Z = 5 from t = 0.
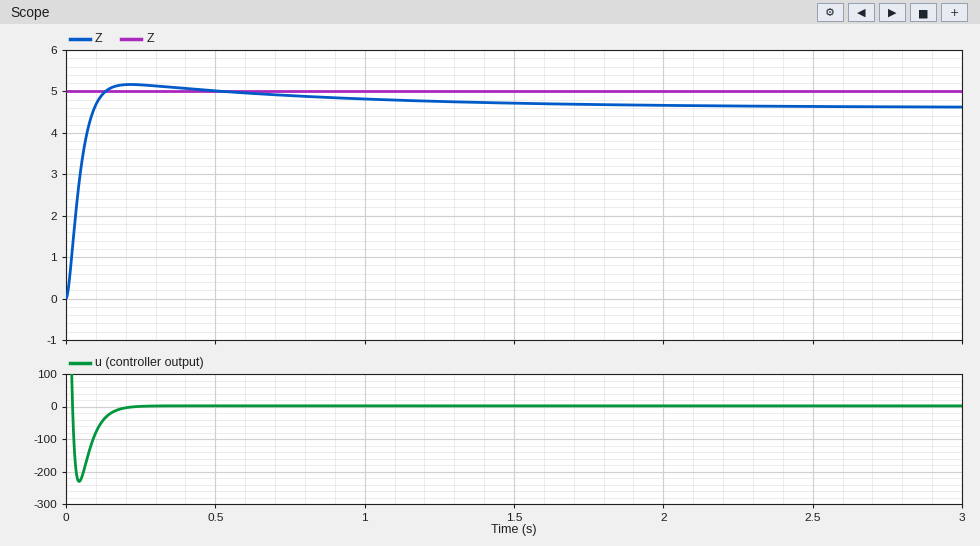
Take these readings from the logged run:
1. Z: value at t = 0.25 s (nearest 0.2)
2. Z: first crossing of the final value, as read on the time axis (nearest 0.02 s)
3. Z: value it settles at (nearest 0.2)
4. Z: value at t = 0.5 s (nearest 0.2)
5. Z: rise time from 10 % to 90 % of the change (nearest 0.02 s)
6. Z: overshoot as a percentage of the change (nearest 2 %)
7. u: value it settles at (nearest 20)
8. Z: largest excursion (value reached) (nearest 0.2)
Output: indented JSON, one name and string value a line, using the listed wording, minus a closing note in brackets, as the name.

{
  "Z: value at t = 0.25 s": "5.2",
  "Z: first crossing of the final value, as read on the time axis": "0.10 s",
  "Z: value it settles at": "4.6",
  "Z: value at t = 0.5 s": "5.0",
  "Z: rise time from 10 % to 90 % of the change": "0.06 s",
  "Z: overshoot as a percentage of the change": "12 %",
  "u: value it settles at": "0",
  "Z: largest excursion (value reached)": "5.2"
}
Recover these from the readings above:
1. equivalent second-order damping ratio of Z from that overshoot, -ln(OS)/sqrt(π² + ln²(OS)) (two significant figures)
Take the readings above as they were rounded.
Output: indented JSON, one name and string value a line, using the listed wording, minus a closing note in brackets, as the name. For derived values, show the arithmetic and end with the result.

{
  "equivalent second-order damping ratio of Z from that overshoot, -ln(OS)/sqrt(π² + ln²(OS))": "ln(0.12) = -2.120; 2.120 / sqrt(9.870 + 4.496) = 0.56"
}
